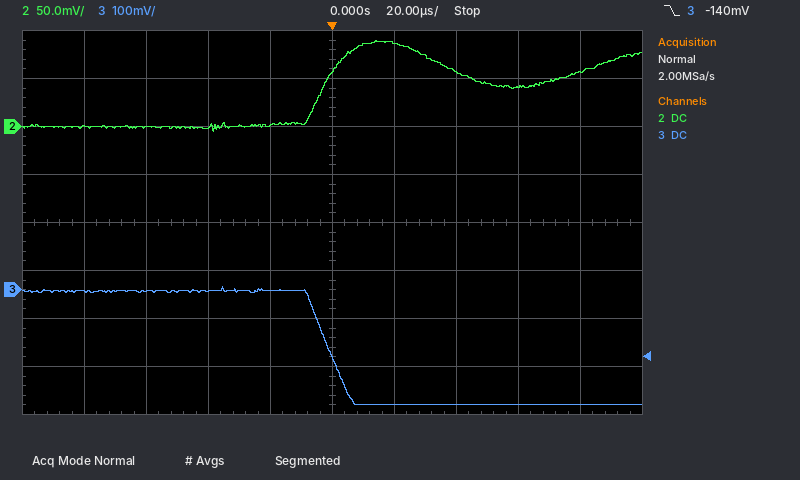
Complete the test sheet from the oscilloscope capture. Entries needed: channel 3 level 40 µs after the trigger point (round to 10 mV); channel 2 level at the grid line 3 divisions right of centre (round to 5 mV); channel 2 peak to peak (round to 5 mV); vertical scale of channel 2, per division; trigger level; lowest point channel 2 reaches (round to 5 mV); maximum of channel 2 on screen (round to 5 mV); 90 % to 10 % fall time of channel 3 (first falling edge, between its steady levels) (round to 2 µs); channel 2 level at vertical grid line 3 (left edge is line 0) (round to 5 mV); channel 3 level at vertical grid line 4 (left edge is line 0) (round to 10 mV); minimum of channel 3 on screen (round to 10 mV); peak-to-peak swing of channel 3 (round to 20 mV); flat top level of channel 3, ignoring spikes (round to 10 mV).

-240 mV
40 mV
95 mV
50 mV
-140 mV
-5 mV
90 mV
12 µs
0 mV
0 mV
-240 mV
240 mV
0 mV
